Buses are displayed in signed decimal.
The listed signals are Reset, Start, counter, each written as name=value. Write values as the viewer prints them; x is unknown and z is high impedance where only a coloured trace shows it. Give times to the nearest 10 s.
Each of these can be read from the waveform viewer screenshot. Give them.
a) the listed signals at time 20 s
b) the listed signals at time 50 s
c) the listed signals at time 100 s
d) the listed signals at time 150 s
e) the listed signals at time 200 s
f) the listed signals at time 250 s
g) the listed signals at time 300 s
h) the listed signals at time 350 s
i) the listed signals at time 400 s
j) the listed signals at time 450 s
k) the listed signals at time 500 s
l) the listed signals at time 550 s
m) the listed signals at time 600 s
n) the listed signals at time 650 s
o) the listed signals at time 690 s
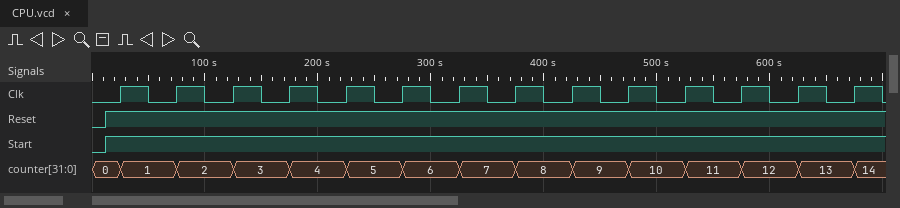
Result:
Reset=1, Start=1, counter=0
Reset=1, Start=1, counter=1
Reset=1, Start=1, counter=2
Reset=1, Start=1, counter=3
Reset=1, Start=1, counter=4
Reset=1, Start=1, counter=5
Reset=1, Start=1, counter=6
Reset=1, Start=1, counter=7
Reset=1, Start=1, counter=8
Reset=1, Start=1, counter=9
Reset=1, Start=1, counter=10
Reset=1, Start=1, counter=11
Reset=1, Start=1, counter=12
Reset=1, Start=1, counter=13
Reset=1, Start=1, counter=14
